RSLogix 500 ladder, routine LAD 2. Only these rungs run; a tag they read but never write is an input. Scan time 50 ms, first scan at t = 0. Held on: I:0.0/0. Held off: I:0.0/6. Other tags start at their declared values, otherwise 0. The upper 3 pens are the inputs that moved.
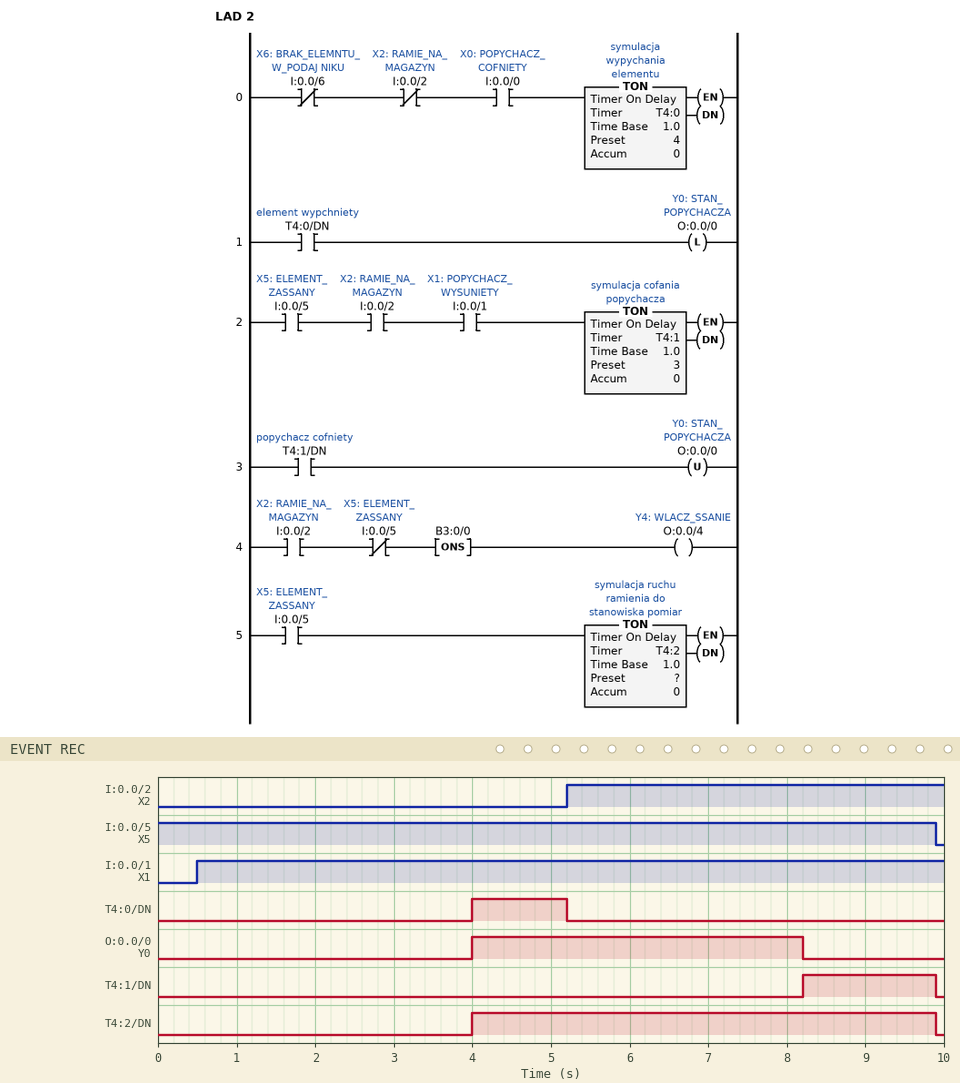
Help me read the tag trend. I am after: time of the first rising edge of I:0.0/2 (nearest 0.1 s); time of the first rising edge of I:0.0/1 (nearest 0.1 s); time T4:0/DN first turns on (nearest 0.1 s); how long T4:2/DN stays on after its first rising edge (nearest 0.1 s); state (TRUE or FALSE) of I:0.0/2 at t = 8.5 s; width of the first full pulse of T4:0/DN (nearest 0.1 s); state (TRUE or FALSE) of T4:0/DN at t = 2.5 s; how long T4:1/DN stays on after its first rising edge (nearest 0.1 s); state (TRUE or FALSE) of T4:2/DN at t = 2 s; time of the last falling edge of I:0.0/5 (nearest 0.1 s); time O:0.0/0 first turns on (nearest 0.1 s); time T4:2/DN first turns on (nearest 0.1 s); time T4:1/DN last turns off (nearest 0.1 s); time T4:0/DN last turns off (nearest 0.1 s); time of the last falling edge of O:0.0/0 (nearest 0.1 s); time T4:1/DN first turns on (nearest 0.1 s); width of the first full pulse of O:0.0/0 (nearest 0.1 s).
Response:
5.2 s
0.5 s
4.0 s
5.9 s
TRUE
1.2 s
FALSE
1.7 s
FALSE
9.9 s
4.0 s
4.0 s
9.9 s
5.2 s
8.2 s
8.2 s
4.2 s
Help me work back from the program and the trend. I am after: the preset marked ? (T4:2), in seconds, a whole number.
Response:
4 s
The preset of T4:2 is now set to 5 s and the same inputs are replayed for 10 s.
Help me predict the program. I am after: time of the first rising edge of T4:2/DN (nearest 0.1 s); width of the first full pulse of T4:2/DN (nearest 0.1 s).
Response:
5.0 s
4.9 s
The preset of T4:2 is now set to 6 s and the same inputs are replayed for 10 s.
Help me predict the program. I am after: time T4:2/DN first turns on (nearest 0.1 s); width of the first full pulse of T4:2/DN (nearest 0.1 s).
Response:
6.0 s
3.9 s
